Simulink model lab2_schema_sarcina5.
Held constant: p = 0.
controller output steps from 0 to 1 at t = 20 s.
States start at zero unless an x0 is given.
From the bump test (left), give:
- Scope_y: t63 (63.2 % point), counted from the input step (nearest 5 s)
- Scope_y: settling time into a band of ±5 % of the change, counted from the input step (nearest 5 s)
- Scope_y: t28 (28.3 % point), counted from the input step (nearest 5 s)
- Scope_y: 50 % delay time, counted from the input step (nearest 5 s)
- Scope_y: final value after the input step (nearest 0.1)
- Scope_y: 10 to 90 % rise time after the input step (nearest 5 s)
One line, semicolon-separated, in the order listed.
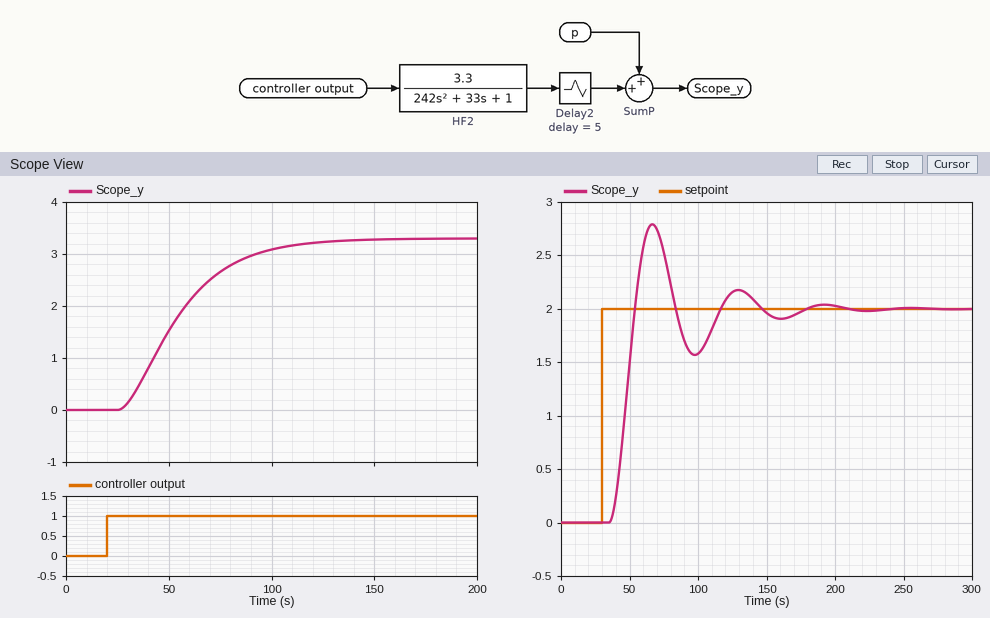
40 s; 85 s; 20 s; 30 s; 3.3; 55 s
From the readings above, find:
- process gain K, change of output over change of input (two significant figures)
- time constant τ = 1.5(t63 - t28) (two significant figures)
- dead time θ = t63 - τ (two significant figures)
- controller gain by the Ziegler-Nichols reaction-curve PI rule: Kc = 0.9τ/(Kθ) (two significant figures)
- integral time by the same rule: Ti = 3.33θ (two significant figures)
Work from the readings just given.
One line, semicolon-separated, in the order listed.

3.3; 30 s; 10 s; 0.82; 33 s
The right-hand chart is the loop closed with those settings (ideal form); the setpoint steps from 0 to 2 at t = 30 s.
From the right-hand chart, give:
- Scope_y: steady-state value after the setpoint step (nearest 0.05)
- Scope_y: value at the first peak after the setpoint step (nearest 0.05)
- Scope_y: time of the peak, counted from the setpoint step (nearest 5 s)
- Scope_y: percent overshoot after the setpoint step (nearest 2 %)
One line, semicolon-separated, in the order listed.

2.00; 2.80; 35 s; 40 %
